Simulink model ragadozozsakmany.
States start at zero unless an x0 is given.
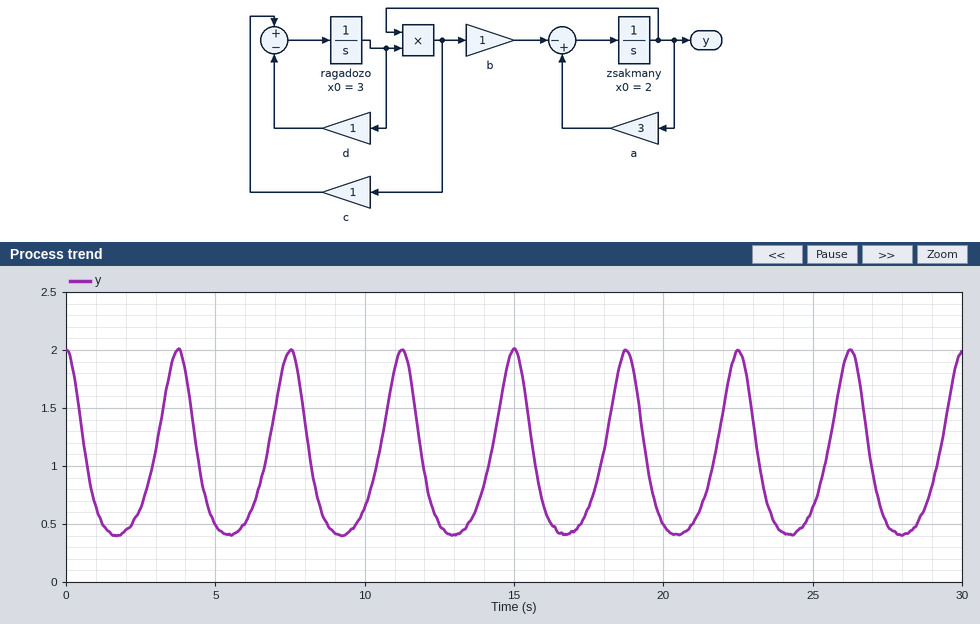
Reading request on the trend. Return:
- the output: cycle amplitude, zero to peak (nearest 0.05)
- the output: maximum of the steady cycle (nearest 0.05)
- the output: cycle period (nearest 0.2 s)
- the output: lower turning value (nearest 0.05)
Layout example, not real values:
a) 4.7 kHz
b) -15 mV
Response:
a) 0.80
b) 2.00
c) 3.8 s
d) 0.40
